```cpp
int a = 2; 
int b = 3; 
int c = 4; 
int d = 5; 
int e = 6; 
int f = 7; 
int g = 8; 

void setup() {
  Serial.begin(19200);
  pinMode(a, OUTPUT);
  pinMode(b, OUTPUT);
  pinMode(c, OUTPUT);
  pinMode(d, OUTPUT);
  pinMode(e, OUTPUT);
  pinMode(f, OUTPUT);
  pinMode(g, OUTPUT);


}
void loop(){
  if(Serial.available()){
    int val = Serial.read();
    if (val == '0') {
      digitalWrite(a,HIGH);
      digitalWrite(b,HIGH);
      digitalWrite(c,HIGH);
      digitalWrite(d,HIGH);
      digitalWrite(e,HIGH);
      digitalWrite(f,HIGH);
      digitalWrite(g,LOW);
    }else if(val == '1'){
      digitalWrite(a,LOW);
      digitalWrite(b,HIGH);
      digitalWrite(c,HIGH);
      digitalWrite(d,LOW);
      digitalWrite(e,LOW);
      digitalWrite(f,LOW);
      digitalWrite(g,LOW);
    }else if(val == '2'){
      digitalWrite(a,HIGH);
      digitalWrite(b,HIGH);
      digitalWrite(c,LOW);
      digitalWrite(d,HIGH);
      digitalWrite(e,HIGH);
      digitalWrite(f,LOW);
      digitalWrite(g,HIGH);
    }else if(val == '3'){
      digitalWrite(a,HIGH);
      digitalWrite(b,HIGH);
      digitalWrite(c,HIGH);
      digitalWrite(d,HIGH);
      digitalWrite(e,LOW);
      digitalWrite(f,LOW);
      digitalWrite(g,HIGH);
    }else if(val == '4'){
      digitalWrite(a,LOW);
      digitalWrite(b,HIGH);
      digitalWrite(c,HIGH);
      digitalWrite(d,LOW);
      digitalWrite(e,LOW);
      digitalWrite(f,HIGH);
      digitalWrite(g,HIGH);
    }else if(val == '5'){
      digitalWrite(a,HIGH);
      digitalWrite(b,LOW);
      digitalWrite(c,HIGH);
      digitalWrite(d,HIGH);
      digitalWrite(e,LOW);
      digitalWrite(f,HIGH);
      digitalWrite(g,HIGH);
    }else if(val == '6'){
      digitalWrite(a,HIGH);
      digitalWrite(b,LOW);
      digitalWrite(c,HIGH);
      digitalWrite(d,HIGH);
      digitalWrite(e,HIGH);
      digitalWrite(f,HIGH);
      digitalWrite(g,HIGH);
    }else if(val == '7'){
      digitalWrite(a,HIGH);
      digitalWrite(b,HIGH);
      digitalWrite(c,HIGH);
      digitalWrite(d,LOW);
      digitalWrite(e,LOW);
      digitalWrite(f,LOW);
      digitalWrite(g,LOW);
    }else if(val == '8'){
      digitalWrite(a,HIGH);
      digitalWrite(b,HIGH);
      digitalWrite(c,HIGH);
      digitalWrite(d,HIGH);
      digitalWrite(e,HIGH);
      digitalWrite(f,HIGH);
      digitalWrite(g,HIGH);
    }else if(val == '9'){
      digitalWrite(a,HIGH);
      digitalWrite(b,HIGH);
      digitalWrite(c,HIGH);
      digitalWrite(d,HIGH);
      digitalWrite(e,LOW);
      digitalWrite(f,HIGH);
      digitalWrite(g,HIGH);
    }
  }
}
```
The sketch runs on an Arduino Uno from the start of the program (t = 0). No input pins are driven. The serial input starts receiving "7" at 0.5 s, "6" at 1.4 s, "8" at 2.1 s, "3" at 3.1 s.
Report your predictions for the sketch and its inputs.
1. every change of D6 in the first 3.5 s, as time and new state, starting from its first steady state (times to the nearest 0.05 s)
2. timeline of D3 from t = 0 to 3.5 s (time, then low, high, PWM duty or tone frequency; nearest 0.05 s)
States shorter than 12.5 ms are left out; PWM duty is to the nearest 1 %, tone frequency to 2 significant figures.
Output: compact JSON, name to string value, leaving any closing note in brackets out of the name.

{"every change of D6 in the first 3.5 s, as time and new state, starting from its first steady state": "0 s low; 1.4 s high; 3.1 s low", "timeline of D3 from t = 0 to 3.5 s": "0 s low; 0.5 s high; 1.4 s low; 2.1 s high"}
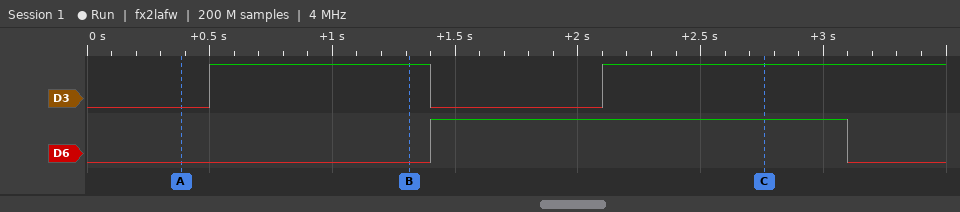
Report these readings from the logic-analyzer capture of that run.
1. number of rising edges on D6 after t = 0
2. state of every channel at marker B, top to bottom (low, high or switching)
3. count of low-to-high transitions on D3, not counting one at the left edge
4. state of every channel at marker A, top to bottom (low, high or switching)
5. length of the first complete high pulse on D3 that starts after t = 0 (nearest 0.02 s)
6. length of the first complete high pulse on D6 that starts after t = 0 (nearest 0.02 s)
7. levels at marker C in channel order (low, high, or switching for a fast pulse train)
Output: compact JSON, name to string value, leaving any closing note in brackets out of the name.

{"number of rising edges on D6 after t = 0": "1", "state of every channel at marker B, top to bottom": "D3 high, D6 low", "count of low-to-high transitions on D3, not counting one at the left edge": "2", "state of every channel at marker A, top to bottom": "D3 low, D6 low", "length of the first complete high pulse on D3 that starts after t = 0": "0.90 s", "length of the first complete high pulse on D6 that starts after t = 0": "1.70 s", "levels at marker C in channel order": "D3 high, D6 high"}
